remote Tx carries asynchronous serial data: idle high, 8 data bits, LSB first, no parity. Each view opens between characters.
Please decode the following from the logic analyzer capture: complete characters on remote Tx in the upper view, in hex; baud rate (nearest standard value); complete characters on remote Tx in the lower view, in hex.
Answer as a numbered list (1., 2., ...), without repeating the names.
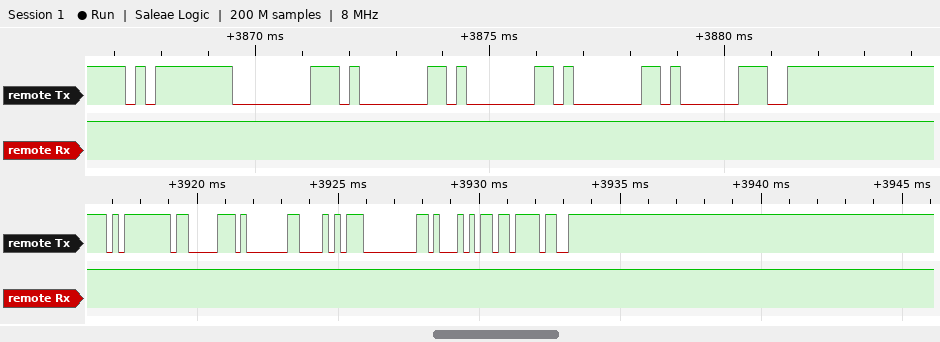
1. FD, 80, 01, 01, 01, 81, FE
2. 4800 baud
3. FD, 83, 01, A8, 00, 51, 7B, FE
